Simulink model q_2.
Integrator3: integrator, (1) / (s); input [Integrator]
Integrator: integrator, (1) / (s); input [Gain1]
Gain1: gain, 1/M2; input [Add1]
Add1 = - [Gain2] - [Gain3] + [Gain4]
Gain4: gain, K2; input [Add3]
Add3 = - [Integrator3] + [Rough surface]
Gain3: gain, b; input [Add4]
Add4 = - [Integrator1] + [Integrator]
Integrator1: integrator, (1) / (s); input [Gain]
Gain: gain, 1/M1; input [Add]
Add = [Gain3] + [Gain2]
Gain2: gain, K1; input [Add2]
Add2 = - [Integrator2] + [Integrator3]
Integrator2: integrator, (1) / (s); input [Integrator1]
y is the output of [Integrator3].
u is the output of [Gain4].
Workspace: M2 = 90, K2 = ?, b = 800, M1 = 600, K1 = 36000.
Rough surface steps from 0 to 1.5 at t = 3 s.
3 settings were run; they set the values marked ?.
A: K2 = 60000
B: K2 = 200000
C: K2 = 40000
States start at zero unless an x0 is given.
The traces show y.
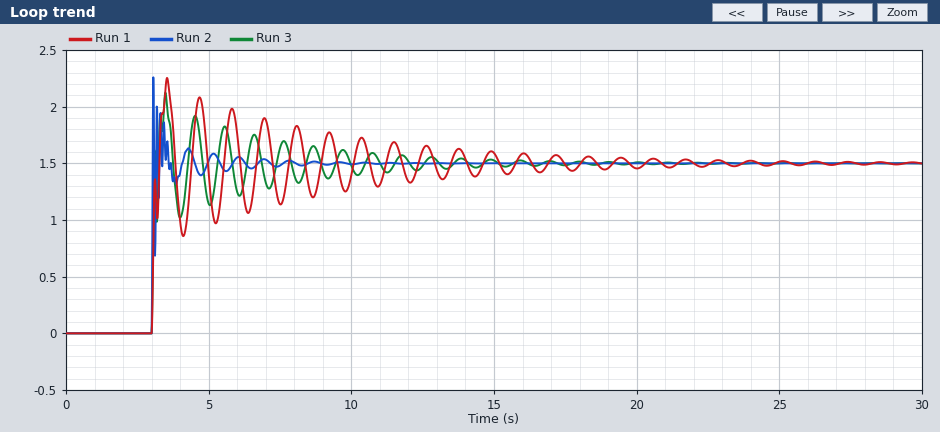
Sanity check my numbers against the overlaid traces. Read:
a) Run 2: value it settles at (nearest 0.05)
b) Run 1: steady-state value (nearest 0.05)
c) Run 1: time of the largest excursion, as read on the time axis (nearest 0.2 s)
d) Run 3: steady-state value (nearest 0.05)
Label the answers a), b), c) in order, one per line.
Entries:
a) 1.50
b) 1.50
c) 3.6 s
d) 1.50
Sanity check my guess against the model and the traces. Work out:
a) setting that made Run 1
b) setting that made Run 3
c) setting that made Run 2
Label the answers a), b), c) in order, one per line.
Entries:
a) C
b) A
c) B
